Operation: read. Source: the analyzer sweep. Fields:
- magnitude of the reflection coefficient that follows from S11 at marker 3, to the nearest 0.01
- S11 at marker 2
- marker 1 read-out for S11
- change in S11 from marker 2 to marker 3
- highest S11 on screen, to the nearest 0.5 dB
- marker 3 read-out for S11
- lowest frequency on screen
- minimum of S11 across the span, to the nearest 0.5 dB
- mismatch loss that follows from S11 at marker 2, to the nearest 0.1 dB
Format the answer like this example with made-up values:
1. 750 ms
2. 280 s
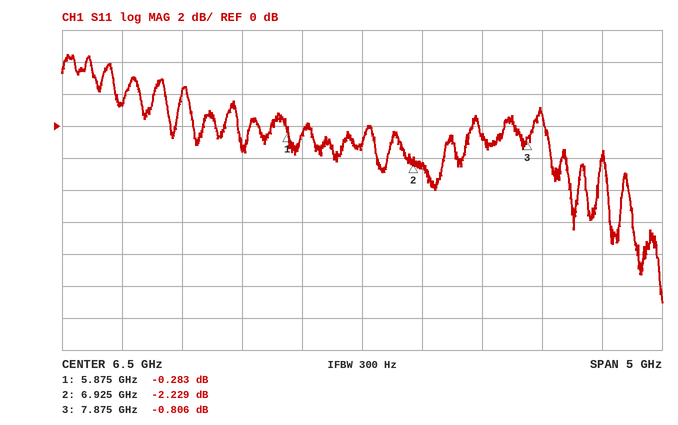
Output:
1. 0.91
2. -2.229 dB
3. -0.283 dB
4. 1.423 dB
5. 4.5 dB
6. -0.806 dB
7. 4 GHz
8. -11.0 dB
9. 4.0 dB
